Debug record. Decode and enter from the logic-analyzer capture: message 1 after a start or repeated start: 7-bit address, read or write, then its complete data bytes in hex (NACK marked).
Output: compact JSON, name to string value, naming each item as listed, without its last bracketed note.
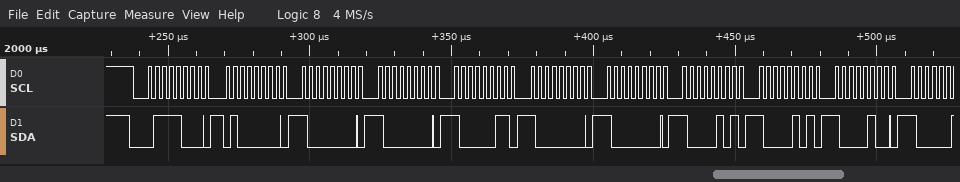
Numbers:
{"message 1 after a start or repeated start: 7-bit address, read or write, then its complete data bytes in hex": "0x3C write: 40 80 80 83 80 80 85 85 84"}
